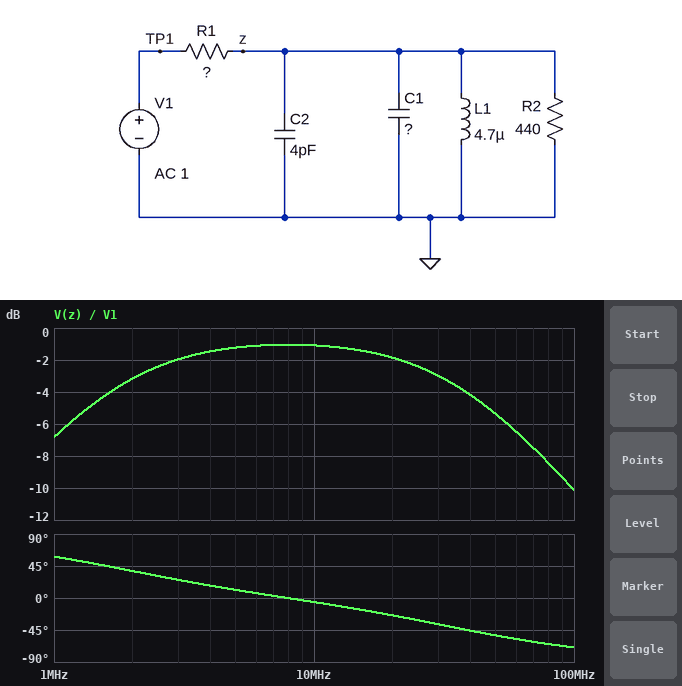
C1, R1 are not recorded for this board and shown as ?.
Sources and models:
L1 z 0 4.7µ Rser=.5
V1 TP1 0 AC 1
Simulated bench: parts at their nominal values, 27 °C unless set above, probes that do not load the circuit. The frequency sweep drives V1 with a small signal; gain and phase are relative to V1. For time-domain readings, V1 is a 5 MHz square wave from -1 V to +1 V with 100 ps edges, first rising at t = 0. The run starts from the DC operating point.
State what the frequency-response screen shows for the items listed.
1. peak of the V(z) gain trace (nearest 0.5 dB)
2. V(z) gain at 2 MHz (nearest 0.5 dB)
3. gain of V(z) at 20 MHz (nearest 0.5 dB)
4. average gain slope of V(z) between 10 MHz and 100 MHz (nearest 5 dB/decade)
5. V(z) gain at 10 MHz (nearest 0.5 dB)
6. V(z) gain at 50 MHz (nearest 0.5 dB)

-1.0 dB
-3.0 dB
-2.0 dB
-10 dB/decade
-1.0 dB
-5.5 dB
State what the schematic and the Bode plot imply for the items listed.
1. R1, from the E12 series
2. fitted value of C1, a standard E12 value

56 Ω
82 pF
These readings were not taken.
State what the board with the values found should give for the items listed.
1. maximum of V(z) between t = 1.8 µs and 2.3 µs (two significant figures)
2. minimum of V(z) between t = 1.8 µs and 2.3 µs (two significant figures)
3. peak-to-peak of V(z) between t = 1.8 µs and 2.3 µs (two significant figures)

1.2 V
-1.2 V
2.4 V
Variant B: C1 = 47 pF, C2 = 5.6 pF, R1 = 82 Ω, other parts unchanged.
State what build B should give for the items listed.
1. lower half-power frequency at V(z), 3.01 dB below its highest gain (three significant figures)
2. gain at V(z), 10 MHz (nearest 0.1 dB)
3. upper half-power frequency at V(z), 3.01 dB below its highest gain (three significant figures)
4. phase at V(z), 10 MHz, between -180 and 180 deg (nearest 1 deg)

2.24 MHz
-1.5 dB
46.0 MHz
0 deg
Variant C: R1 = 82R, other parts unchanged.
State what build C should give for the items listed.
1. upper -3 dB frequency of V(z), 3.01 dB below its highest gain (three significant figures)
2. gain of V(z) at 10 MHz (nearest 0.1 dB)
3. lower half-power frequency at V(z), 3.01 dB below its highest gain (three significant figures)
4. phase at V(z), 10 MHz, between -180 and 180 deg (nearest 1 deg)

29.0 MHz
-1.6 dB
2.18 MHz
-8 deg
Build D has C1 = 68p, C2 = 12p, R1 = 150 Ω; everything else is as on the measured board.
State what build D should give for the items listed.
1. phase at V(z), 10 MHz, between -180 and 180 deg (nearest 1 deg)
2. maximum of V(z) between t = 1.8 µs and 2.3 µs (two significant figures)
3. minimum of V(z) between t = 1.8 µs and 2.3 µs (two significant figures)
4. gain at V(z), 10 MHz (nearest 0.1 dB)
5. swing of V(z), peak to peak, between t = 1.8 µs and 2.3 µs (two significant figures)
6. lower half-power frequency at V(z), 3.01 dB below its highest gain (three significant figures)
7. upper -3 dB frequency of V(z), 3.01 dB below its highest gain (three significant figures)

-10 deg
1.1 V
-1.1 V
-2.7 dB
2.1 V
3.22 MHz
21.0 MHz
